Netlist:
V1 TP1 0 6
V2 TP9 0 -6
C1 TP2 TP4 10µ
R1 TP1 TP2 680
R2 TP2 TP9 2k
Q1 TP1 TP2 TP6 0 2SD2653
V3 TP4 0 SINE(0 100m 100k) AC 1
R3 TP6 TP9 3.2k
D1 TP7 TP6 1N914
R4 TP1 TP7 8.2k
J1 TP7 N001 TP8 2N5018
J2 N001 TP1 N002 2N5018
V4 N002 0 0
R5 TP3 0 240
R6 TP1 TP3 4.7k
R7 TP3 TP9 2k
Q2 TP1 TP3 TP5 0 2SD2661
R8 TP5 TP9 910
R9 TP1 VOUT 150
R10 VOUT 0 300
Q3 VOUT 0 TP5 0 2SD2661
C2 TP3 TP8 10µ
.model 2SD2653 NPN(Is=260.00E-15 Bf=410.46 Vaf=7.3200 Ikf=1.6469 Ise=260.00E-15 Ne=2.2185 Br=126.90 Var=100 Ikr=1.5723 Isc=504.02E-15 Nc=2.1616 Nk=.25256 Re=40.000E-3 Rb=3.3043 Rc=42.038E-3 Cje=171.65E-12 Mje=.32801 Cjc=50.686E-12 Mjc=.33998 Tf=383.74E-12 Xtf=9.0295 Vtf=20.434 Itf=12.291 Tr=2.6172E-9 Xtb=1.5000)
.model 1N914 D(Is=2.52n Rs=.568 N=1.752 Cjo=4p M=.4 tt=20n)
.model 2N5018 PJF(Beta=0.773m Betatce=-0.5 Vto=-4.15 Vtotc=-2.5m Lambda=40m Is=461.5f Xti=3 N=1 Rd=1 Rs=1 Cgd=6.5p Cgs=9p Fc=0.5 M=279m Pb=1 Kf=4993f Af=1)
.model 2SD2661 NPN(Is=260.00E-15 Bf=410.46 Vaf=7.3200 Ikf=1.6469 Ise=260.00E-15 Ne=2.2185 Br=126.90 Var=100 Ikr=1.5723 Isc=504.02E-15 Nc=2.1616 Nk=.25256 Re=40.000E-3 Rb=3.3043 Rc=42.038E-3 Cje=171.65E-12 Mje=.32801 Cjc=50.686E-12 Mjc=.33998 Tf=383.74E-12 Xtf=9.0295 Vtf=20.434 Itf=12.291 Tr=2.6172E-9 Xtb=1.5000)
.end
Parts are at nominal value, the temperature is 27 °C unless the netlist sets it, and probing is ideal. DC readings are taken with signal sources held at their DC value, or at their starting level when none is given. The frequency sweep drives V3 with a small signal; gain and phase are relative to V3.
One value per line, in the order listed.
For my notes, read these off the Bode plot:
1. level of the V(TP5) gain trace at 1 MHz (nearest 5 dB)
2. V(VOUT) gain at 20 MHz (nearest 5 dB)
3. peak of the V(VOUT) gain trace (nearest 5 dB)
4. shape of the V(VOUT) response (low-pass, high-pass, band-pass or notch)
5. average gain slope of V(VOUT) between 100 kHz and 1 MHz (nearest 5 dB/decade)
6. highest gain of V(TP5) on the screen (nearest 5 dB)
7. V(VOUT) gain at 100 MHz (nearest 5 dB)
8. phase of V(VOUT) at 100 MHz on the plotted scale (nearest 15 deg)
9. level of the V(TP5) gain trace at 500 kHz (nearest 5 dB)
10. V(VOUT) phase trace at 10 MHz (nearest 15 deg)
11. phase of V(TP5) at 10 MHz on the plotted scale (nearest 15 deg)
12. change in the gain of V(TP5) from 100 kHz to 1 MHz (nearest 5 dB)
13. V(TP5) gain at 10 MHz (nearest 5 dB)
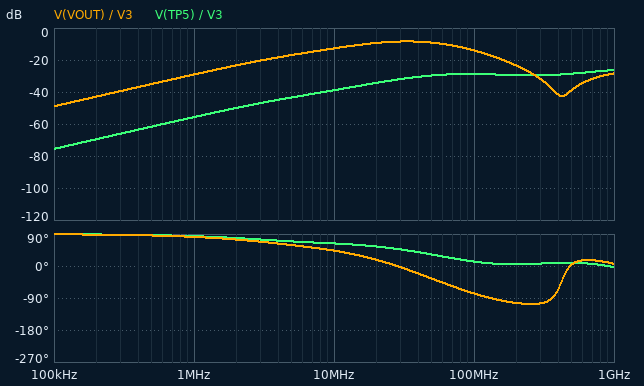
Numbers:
-55 dB
-10 dB
-10 dB
band-pass
20 dB/decade
-25 dB
-15 dB
-75 deg
-60 dB
45 deg
60 deg
20 dB
-40 dB
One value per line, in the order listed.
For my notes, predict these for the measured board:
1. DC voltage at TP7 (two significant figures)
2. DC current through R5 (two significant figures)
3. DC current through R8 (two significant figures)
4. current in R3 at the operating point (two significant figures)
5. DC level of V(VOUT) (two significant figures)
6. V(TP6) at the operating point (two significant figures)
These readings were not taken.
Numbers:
2.9 V
1.5 mA
5.9 mA
2.6 mA
3.4 V
2.4 V
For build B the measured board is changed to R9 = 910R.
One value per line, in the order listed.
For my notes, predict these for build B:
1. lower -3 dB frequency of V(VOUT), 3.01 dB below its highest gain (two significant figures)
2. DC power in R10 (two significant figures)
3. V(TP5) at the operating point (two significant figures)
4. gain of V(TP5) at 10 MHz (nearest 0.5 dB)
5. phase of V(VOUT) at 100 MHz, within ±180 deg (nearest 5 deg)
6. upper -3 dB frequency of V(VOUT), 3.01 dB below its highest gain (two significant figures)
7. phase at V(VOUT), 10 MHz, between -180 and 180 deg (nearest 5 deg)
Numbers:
5.9 MHz
81 µW
-620 mV
-37.0 dB
-95 deg
42 MHz
20 deg
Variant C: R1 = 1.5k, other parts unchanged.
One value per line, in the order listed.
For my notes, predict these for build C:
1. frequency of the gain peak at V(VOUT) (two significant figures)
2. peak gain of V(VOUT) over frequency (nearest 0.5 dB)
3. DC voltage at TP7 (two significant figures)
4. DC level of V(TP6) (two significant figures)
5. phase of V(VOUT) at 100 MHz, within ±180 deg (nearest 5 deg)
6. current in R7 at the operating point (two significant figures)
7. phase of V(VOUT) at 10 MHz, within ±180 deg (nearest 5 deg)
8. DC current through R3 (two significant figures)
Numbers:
21 MHz
-10.5 dB
850 mV
290 mV
-90 deg
2.8 mA
25 deg
2.0 mA
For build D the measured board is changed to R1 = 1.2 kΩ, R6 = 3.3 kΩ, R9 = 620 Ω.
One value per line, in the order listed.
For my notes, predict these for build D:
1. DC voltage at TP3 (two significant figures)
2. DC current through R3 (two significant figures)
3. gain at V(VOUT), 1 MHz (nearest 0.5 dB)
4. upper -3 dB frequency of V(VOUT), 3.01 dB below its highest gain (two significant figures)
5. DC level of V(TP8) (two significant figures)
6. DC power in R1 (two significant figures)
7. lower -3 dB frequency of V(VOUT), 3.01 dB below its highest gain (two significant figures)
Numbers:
-240 mV
2.2 mA
-19.0 dB
33 MHz
1.5 V
17 mW
4.5 MHz
